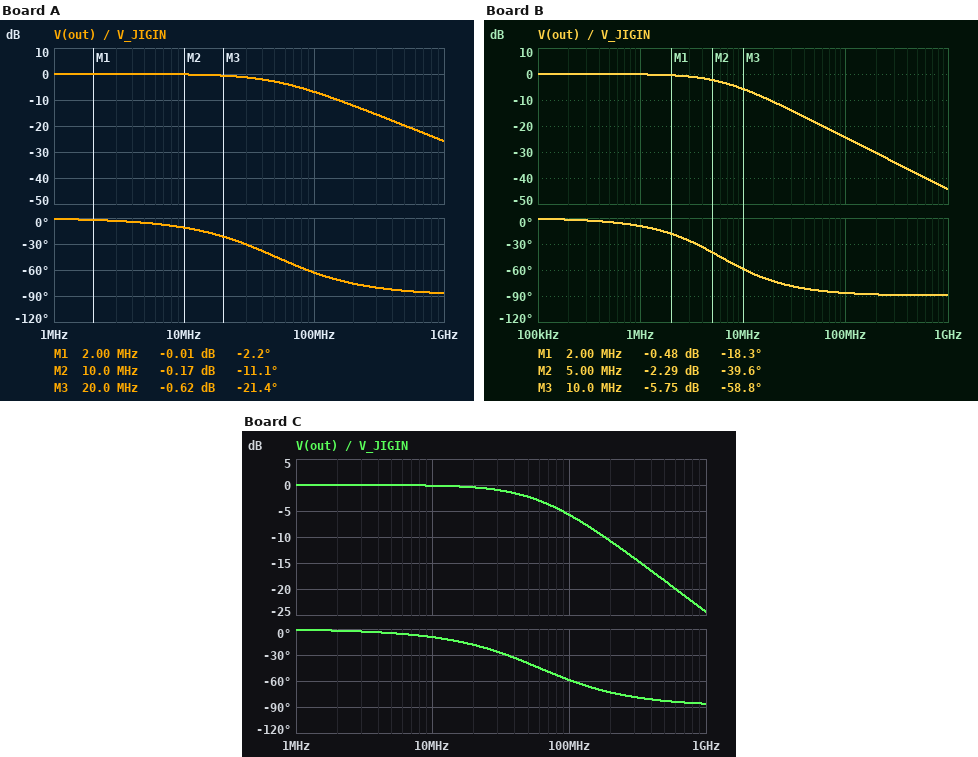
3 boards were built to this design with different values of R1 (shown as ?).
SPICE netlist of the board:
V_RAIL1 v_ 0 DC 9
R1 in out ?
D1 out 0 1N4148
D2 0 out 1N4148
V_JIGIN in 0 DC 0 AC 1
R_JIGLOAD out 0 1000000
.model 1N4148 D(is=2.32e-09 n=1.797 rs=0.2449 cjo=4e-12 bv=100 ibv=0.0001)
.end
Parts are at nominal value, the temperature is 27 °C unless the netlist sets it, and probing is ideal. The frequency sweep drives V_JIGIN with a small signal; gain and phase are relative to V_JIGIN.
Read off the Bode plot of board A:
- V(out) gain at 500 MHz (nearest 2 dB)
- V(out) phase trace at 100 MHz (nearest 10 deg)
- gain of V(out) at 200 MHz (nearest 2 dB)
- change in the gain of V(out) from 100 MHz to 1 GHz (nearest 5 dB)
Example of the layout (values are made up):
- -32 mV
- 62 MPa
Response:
- -20 dB
- -60 deg
- -12 dB
- -20 dB
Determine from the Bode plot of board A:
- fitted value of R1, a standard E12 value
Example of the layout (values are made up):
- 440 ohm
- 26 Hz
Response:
- 390 Ω
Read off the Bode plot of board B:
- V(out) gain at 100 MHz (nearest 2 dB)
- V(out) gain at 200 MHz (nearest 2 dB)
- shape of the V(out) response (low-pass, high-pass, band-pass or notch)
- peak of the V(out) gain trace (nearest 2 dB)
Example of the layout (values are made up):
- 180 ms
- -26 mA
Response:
- -24 dB
- -30 dB
- low-pass
- 0 dB
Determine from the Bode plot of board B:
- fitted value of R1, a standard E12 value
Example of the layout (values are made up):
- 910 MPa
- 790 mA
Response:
- 3.3 kΩ
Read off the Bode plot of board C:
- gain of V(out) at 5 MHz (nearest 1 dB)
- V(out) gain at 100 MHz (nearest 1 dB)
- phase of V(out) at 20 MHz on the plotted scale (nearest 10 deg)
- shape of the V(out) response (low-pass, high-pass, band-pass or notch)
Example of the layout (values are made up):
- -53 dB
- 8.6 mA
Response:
- 0 dB
- -6 dB
- -20 deg
- low-pass
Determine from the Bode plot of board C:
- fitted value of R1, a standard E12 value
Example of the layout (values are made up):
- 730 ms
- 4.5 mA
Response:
- 330 Ω
